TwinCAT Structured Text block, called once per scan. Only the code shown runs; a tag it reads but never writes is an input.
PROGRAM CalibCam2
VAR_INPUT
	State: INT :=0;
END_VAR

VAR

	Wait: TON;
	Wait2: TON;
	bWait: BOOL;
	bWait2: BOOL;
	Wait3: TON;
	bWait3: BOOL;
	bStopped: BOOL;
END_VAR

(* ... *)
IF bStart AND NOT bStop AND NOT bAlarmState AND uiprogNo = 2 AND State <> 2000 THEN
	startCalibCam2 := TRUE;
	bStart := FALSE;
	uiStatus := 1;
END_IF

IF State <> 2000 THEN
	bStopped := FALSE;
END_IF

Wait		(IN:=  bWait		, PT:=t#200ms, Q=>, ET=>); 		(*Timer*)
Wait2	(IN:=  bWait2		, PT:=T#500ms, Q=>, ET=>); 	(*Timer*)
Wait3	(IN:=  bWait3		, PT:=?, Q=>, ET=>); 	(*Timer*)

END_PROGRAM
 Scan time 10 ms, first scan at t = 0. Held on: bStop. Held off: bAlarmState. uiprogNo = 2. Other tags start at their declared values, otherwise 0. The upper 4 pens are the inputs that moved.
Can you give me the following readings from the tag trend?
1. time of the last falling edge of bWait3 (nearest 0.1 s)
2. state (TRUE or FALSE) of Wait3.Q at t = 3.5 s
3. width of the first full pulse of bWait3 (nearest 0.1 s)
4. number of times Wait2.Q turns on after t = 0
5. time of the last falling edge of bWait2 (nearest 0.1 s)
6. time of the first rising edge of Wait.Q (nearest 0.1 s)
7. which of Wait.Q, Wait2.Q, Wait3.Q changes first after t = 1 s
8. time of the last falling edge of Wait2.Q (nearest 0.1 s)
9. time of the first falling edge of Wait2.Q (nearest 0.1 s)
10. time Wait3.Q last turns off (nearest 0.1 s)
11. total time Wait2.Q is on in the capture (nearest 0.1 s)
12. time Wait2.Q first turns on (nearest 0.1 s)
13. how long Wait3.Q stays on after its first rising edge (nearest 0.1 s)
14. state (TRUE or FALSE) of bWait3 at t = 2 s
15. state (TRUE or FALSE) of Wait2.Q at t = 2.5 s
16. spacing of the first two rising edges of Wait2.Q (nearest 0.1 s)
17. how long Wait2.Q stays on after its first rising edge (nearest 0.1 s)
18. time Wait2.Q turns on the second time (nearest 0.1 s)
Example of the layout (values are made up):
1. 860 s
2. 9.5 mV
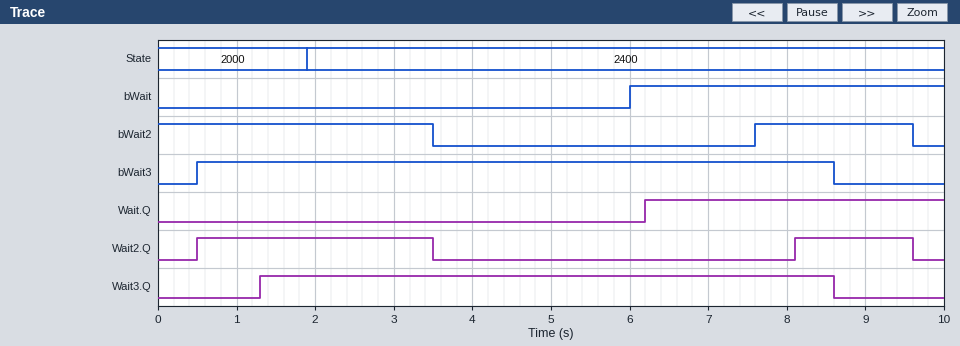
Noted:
1. 8.6 s
2. TRUE
3. 8.1 s
4. 2
5. 9.6 s
6. 6.2 s
7. Wait3.Q
8. 9.6 s
9. 3.5 s
10. 8.6 s
11. 4.5 s
12. 0.5 s
13. 7.3 s
14. TRUE
15. TRUE
16. 7.6 s
17. 3.0 s
18. 8.1 s
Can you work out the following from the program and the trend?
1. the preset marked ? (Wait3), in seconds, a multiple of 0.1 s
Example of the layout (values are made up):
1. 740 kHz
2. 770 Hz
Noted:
1. 0.8 s
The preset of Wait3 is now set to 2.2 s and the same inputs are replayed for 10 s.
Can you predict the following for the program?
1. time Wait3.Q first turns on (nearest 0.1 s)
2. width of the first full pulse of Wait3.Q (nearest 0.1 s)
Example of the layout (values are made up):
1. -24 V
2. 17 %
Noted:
1. 2.7 s
2. 5.9 s
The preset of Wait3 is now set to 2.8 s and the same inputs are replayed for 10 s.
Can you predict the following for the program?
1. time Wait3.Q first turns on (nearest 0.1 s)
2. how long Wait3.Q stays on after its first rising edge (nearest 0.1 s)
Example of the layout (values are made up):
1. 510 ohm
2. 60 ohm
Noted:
1. 3.3 s
2. 5.3 s
